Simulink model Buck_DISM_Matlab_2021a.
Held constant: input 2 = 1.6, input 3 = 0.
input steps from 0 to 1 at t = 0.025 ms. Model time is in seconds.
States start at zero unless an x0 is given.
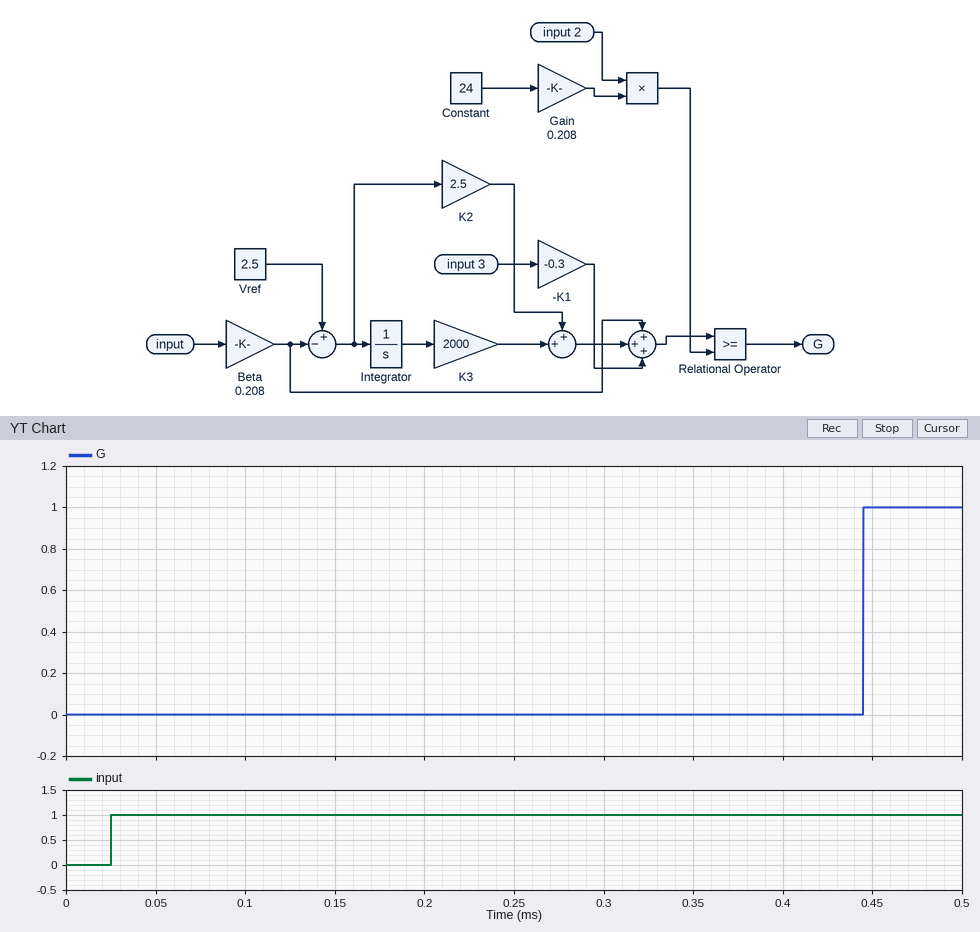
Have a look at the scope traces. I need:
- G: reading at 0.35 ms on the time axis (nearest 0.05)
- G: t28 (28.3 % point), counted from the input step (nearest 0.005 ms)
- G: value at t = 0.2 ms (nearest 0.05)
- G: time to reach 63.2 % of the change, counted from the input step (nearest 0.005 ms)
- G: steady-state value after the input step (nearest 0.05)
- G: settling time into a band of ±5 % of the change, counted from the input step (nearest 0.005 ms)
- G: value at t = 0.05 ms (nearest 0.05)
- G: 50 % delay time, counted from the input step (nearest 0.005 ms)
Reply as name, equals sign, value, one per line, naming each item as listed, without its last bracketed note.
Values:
G: reading at 0.35 ms on the time axis = 0.00
G: t28 (28.3 % point), counted from the input step = 0.420 ms
G: value at t = 0.2 ms = 0.00
G: time to reach 63.2 % of the change, counted from the input step = 0.420 ms
G: steady-state value after the input step = 1.00
G: settling time into a band of ±5 % of the change, counted from the input step = 0.420 ms
G: value at t = 0.05 ms = 0.00
G: 50 % delay time, counted from the input step = 0.420 ms
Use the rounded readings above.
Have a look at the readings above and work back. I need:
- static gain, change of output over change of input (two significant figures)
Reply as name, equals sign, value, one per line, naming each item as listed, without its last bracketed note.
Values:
static gain, change of output over change of input = 1.0
